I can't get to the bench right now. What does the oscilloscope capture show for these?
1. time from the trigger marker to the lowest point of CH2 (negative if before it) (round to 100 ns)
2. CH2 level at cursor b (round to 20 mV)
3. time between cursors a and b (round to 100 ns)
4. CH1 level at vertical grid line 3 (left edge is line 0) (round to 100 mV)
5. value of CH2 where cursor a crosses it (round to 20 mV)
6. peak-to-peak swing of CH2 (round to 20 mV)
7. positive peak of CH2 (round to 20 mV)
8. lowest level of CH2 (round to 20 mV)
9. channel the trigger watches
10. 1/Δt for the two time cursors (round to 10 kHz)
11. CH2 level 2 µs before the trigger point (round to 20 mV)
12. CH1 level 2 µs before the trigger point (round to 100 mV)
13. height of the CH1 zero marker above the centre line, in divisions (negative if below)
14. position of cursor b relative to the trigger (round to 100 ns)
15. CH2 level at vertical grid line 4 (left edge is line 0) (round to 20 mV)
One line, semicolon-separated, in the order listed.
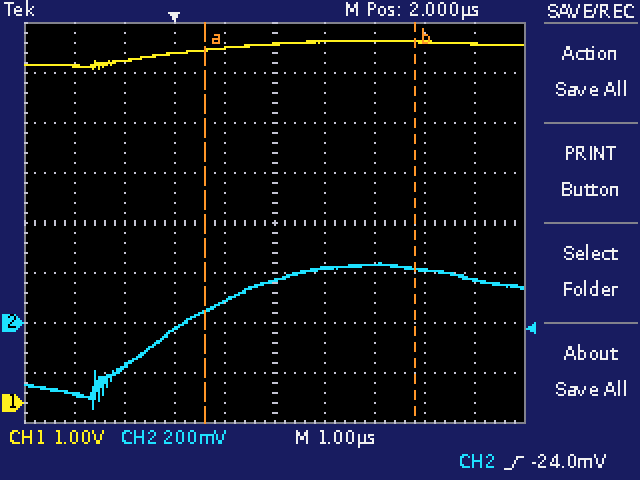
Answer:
-1.6 µs; 220 mV; 4.2 µs; 7.0 V; 40 mV; 580 mV; 240 mV; -340 mV; CH2; 240 kHz; -280 mV; 6.7 V; -3.6 div; +4.8 µs; 80 mV
